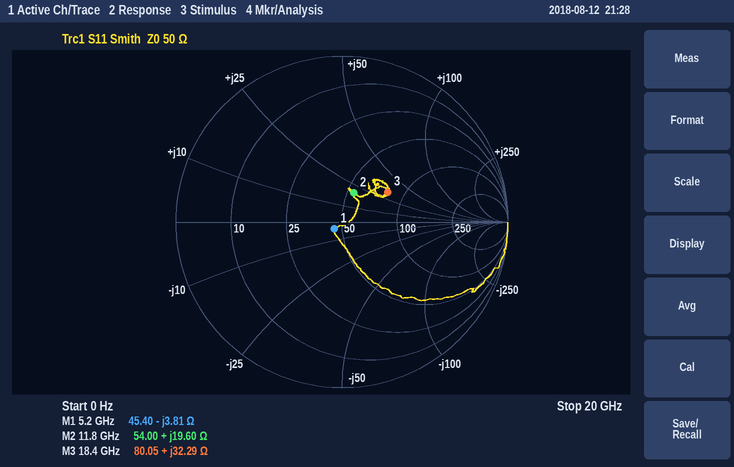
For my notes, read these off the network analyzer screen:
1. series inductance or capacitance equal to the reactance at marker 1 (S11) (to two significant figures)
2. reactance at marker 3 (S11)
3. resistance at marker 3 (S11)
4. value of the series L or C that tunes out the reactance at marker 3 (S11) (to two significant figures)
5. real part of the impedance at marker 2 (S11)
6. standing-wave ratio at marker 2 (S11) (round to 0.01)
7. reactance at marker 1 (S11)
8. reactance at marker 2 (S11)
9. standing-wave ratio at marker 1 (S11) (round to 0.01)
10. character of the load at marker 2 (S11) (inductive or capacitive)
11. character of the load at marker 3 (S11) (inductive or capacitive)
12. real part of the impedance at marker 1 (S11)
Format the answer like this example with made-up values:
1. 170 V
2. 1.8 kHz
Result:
1. 8.0 pF
2. +32.29 Ω
3. 80.05 Ω
4. 270 fF
5. 54.00 Ω
6. 1.47
7. -3.81 Ω
8. +19.60 Ω
9. 1.13
10. inductive
11. inductive
12. 45.40 Ω
